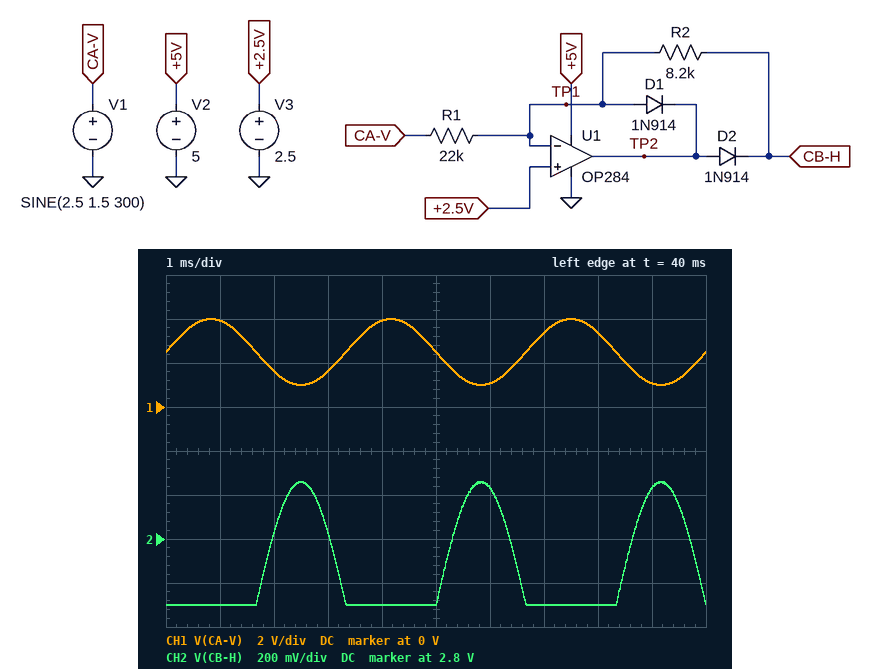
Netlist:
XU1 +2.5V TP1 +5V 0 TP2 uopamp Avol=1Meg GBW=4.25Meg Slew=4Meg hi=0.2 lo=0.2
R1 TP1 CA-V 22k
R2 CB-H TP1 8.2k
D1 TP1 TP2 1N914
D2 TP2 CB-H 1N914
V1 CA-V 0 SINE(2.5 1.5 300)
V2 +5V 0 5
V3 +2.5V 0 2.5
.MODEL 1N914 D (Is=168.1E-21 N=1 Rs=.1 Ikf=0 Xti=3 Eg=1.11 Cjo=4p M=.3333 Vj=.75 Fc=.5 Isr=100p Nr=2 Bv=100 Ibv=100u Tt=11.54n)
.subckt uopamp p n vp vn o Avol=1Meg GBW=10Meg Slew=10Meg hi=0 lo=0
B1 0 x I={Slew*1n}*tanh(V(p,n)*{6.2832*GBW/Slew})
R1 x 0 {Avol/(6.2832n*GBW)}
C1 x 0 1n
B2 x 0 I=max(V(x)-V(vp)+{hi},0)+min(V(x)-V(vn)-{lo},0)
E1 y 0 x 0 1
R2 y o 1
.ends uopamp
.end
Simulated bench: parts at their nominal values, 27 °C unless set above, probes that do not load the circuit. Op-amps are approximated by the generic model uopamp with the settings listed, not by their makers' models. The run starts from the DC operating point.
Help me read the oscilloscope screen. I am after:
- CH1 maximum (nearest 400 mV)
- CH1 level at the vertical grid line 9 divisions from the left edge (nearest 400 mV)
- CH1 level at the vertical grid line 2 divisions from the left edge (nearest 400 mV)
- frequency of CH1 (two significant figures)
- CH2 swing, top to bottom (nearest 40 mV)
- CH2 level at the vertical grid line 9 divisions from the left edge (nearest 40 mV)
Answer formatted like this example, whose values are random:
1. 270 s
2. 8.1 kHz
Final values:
1. 4.0 V
2. 1.2 V
3. 1.6 V
4. 300 Hz
5. 560 mV
6. 3.04 V
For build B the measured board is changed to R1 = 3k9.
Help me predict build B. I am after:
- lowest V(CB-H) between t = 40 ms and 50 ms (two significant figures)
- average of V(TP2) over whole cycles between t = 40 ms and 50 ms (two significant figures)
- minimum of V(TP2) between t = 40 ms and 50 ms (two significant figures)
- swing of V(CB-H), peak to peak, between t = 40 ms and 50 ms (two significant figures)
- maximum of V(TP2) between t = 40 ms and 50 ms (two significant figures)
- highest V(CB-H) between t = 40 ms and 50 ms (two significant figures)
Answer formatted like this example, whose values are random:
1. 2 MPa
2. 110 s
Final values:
1. 2.5 V
2. 3.1 V
3. 1.7 V
4. 1.5 V
5. 4.8 V
6. 4.0 V
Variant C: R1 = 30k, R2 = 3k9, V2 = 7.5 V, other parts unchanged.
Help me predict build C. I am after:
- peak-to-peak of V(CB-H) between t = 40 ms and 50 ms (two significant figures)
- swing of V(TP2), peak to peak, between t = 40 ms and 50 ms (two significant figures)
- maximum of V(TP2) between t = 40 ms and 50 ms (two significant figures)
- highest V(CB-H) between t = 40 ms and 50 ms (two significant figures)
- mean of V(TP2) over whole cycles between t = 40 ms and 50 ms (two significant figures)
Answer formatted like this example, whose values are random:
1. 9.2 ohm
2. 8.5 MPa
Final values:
1. 200 mV
2. 1.6 V
3. 3.4 V
4. 2.7 V
5. 2.6 V
